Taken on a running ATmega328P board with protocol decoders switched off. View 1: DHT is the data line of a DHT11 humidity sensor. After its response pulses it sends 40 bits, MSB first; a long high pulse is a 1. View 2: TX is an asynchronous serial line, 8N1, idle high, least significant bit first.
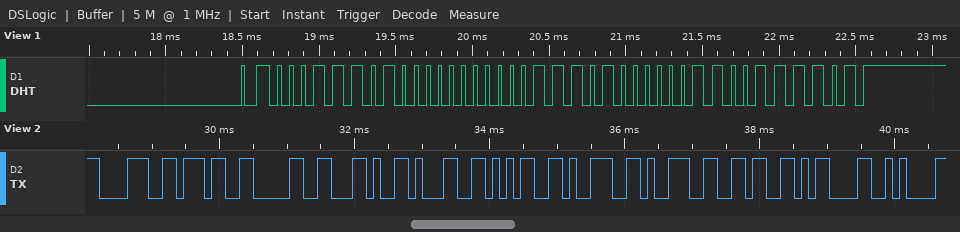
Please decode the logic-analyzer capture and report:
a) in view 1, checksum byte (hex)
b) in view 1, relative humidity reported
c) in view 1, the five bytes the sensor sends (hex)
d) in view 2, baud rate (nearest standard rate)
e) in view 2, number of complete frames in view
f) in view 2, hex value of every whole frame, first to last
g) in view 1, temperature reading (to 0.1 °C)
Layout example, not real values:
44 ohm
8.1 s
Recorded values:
0x3D
29 %
1D 00 1D 03 3D
9600 baud
11
38 37 30 2C 31 35 39 39 36 0D 0A
29.3 °C
